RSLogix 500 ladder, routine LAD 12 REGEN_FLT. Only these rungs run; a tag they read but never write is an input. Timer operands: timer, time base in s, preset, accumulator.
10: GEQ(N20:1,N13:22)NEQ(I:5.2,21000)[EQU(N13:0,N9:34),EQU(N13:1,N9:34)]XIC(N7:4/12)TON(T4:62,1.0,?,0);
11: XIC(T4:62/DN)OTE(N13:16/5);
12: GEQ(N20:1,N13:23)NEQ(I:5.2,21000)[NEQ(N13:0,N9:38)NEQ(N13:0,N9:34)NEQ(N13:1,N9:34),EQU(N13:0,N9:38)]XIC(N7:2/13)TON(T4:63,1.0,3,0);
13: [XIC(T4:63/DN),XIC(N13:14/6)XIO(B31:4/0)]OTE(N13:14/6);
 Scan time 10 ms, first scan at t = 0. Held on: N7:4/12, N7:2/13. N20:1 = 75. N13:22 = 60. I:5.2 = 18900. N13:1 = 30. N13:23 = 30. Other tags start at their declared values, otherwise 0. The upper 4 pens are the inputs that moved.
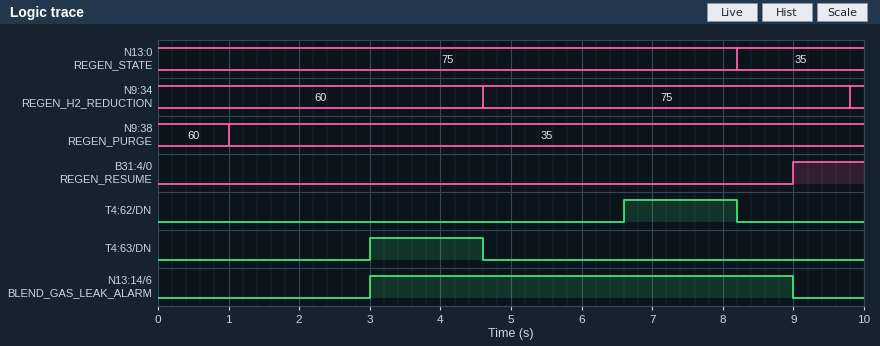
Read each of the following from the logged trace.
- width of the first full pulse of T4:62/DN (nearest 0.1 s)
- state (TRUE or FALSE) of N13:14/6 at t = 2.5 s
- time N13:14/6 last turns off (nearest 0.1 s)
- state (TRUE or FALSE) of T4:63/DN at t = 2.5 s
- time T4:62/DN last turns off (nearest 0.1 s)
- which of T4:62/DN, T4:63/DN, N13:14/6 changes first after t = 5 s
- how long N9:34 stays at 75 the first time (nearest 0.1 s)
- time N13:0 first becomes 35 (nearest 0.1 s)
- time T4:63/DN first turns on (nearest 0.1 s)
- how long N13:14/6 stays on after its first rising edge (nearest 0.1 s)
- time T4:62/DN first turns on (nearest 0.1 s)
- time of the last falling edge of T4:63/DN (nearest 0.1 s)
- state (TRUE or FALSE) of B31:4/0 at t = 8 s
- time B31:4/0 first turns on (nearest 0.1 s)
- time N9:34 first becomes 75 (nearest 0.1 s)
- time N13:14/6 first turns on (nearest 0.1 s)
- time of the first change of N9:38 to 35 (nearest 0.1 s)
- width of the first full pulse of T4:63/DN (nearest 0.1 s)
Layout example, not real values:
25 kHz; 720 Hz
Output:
1.6 s; FALSE; 9.0 s; FALSE; 8.2 s; T4:62/DN; 5.2 s; 8.2 s; 3.0 s; 6.0 s; 6.6 s; 4.6 s; FALSE; 9.0 s; 4.6 s; 3.0 s; 1.0 s; 1.6 s
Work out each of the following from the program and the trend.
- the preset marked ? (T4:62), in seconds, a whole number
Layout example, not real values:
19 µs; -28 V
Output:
2 s
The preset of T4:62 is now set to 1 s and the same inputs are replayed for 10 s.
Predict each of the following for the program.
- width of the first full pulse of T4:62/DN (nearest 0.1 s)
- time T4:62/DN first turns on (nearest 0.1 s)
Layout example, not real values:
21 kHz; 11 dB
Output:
2.6 s; 5.6 s
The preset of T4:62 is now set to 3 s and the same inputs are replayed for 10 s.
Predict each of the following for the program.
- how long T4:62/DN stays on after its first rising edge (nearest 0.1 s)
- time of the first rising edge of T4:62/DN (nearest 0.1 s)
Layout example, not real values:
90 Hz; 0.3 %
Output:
0.6 s; 7.6 s
